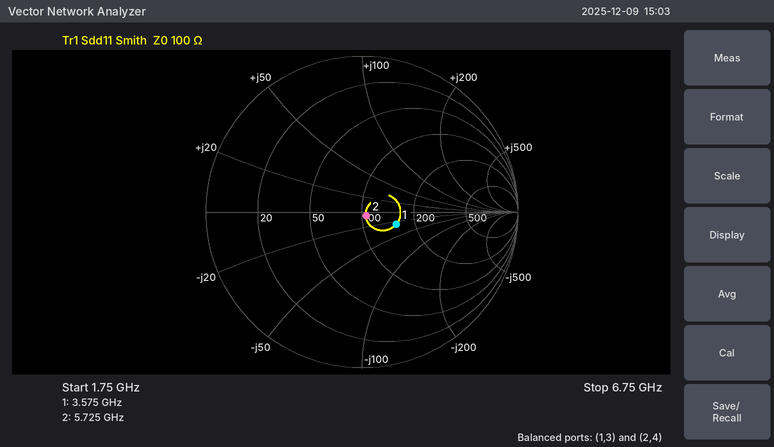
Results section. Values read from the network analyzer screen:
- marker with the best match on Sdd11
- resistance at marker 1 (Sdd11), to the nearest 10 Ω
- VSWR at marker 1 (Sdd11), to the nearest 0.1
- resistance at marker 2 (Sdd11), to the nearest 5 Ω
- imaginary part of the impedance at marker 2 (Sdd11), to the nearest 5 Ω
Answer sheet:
marker 2
150 Ω
1.6
105 Ω
-5 Ω
